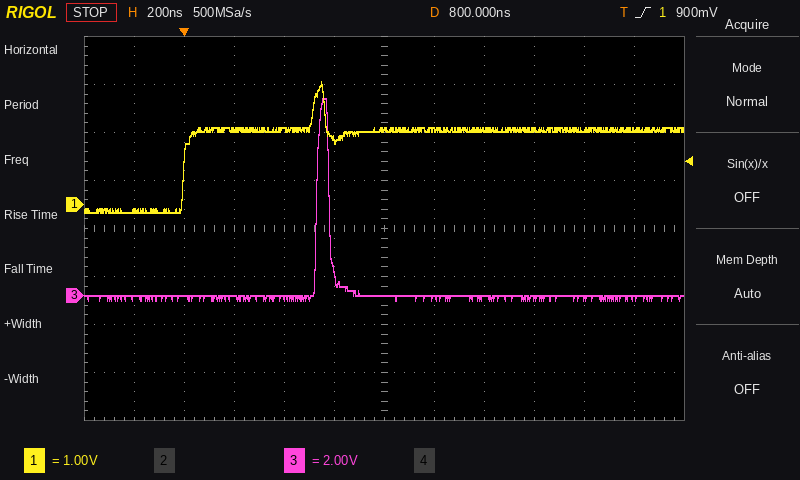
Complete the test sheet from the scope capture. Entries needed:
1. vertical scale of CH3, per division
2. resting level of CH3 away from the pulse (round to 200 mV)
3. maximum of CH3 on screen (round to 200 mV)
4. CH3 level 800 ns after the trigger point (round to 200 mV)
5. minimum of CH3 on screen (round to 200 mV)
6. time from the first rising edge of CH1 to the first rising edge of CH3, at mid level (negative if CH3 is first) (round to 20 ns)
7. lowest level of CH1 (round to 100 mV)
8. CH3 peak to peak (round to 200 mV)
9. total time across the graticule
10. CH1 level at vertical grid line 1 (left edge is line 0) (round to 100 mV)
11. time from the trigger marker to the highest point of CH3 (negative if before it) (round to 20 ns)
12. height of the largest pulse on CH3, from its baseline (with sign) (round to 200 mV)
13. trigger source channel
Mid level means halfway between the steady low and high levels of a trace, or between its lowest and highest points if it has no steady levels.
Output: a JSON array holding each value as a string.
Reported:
["2 V", "0.0 V", "8.2 V", "0.0 V", "-200 mV", "+540 ns", "-200 mV", "8.4 V", "2.4 µs", "-100 mV", "+560 ns", "+8.2 V", "CH1"]
